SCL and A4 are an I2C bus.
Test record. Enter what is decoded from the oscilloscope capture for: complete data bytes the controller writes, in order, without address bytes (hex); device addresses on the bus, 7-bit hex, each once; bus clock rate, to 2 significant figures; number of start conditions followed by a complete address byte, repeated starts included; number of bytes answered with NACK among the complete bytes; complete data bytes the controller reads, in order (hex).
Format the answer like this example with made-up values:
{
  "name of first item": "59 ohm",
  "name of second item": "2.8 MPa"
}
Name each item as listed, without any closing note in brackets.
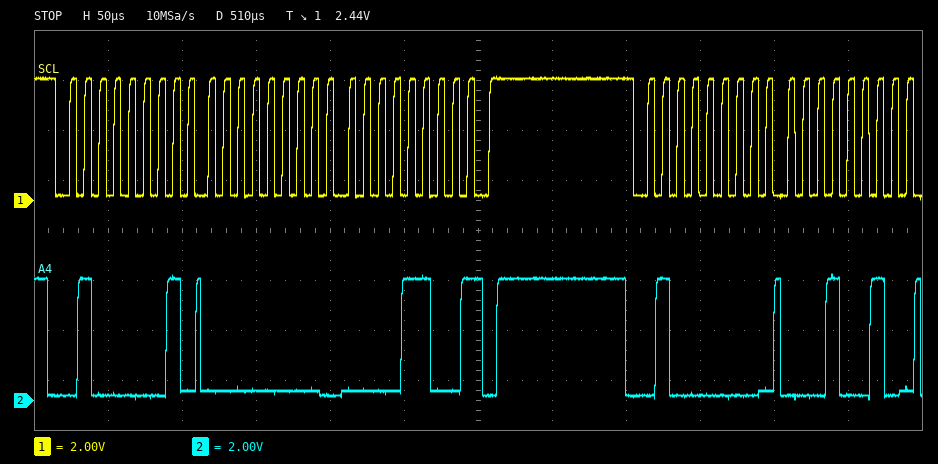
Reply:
{
  "complete data bytes the controller writes, in order, without address bytes": "12",
  "device addresses on the bus, 7-bit hex, each once": "0x20",
  "bus clock rate, to 2 significant figures": "100 kHz",
  "number of start conditions followed by a complete address byte, repeated starts included": "2",
  "number of bytes answered with NACK among the complete bytes": "1",
  "complete data bytes the controller reads, in order": "00 0C"
}
